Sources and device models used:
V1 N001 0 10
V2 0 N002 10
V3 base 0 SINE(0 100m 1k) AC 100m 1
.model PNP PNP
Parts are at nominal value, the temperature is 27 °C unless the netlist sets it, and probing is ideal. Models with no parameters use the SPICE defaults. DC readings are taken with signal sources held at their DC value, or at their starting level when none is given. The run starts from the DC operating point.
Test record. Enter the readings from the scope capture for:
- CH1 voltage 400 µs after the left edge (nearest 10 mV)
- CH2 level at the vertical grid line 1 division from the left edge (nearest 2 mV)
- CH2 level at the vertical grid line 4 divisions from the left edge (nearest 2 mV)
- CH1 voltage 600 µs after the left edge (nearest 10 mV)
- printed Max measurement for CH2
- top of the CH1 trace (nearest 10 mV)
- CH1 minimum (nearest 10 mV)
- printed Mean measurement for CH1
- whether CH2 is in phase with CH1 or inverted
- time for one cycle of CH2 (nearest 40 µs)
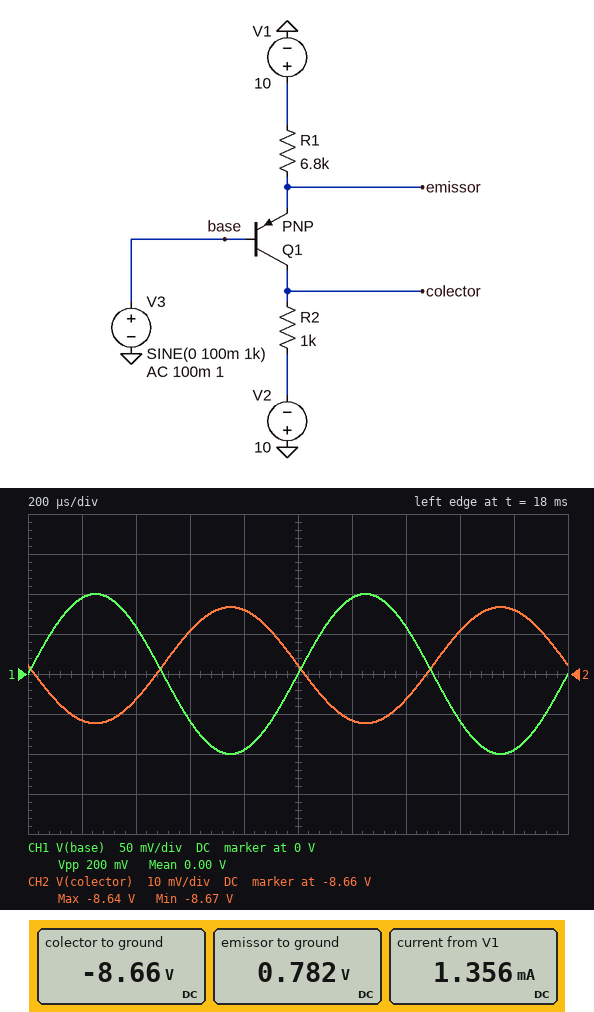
60 mV
-8.672 V
-8.644 V
-60 mV
-8.64 V
100 mV
-100 mV
0.00 V
inverted
1.00 ms
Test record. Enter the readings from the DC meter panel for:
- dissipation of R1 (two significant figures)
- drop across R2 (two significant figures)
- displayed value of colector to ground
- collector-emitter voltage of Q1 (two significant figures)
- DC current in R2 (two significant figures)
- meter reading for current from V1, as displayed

12 mW
1.3 V
-8.66 V
-9.4 V
1.3 mA
1.356 mA
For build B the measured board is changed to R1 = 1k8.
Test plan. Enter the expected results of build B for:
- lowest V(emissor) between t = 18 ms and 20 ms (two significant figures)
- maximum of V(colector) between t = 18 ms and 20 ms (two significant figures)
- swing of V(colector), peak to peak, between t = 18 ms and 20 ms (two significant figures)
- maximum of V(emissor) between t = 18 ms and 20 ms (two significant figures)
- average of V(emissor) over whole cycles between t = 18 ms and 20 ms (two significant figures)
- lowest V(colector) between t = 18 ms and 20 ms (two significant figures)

720 mV
-4.9 V
110 mV
920 mV
820 mV
-5.0 V
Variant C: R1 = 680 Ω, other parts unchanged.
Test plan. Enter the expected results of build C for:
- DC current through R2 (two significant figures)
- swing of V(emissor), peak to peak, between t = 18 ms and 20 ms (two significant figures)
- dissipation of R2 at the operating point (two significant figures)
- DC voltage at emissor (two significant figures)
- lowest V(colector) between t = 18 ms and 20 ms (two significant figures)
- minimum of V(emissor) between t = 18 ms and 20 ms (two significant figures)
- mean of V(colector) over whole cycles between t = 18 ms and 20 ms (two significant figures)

11 mA
200 mV
120 mW
850 mV
700 mV
750 mV
800 mV
